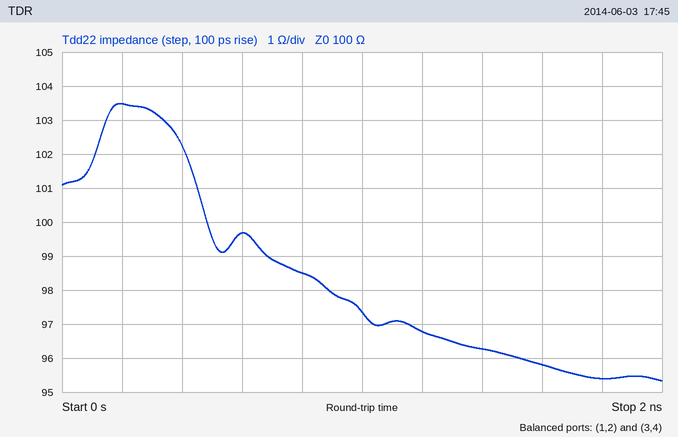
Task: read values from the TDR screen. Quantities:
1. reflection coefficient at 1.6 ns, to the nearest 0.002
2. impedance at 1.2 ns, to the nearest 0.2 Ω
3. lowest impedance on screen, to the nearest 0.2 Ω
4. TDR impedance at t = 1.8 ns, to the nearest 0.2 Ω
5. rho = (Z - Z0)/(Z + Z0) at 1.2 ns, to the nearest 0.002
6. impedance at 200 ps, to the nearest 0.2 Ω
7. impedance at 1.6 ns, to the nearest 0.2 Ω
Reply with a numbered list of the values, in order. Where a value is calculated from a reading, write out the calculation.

1. (95.8 − 100)/(95.8 + 100) ≈ -0.022
2. 96.8 Ω
3. 95.4 Ω
4. 95.4 Ω
5. (96.8 − 100)/(96.8 + 100) ≈ -0.016
6. 103.4 Ω
7. 95.8 Ω
